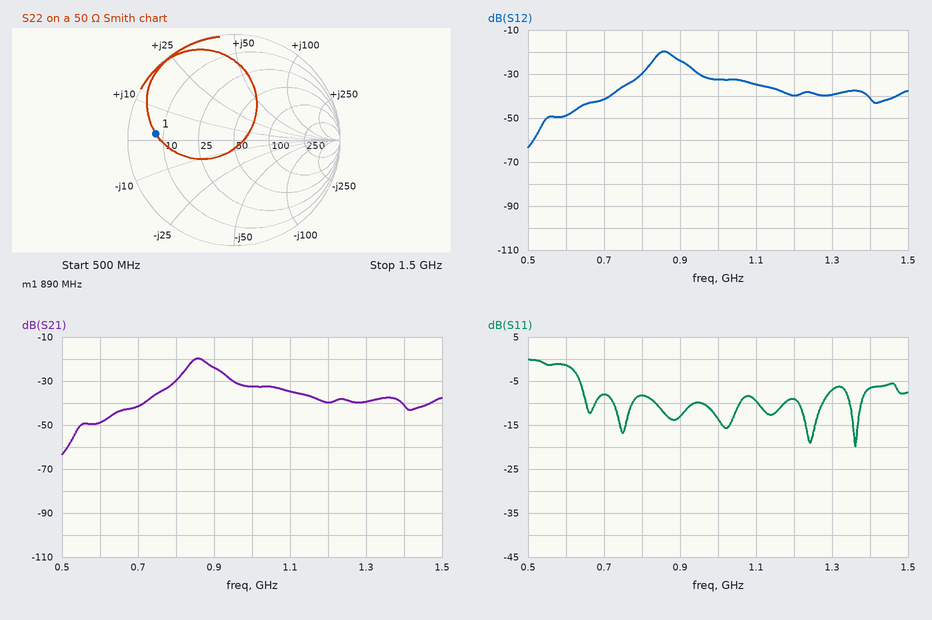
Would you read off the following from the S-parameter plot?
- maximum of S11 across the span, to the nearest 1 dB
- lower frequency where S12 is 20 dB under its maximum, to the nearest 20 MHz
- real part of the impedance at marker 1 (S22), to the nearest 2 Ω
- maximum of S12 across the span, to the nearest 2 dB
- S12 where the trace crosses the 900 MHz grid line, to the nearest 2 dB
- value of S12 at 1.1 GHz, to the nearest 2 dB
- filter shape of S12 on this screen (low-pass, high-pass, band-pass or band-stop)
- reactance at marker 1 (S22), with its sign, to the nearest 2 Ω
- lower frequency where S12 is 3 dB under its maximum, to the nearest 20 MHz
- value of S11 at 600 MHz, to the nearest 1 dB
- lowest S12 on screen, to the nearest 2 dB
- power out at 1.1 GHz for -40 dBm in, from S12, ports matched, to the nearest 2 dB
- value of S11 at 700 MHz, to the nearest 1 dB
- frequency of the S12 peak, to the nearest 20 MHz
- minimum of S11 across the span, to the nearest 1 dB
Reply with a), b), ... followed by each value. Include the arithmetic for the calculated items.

a) 0 dB
b) 720 MHz
c) 8 Ω
d) -20 dB
e) -24 dB
f) -34 dB
g) band-pass
h) +2 Ω
i) 840 MHz
j) -1 dB
k) -64 dB
l) -40 dBm + (-34 dB) = -74 dBm
m) -8 dB
n) 860 MHz
o) -20 dB
